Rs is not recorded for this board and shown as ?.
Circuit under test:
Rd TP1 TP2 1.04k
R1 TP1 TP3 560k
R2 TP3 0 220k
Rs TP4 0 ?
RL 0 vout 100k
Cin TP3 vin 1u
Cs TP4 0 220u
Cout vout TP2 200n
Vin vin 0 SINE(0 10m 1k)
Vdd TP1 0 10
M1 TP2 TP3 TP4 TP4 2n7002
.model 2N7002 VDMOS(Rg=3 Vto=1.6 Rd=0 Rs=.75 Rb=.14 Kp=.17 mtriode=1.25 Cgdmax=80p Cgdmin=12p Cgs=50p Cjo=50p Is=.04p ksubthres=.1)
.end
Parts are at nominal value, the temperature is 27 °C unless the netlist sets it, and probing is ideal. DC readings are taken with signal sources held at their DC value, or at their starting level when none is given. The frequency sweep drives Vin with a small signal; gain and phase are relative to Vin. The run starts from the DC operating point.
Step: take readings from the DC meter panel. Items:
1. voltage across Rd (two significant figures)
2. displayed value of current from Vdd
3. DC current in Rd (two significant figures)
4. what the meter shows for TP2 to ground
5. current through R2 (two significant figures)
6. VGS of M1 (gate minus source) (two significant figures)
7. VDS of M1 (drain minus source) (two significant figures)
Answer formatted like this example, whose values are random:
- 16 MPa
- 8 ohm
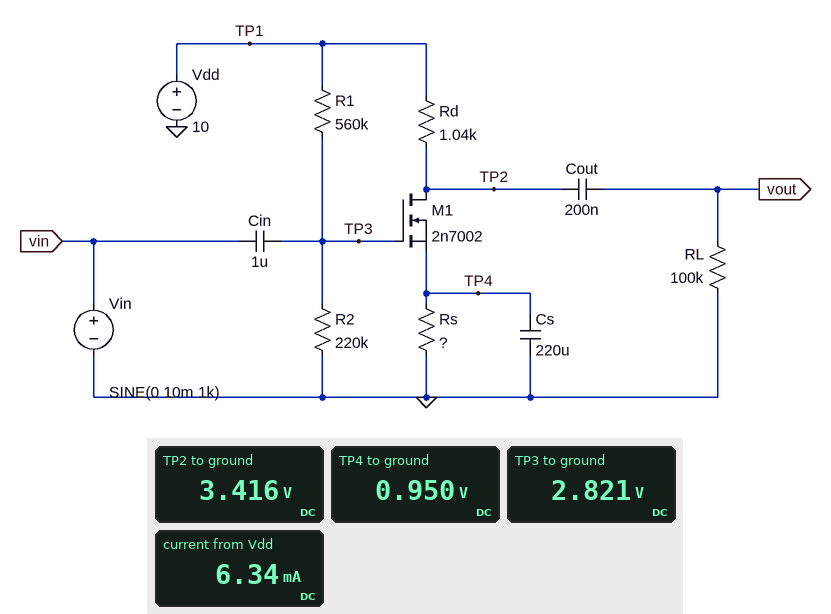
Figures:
- 6.6 V
- 6.34 mA
- 6.3 mA
- 3.416 V
- 13 µA
- 1.9 V
- 2.5 V
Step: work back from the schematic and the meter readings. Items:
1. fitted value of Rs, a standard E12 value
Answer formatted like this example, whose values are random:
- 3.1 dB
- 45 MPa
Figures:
- 150 Ω
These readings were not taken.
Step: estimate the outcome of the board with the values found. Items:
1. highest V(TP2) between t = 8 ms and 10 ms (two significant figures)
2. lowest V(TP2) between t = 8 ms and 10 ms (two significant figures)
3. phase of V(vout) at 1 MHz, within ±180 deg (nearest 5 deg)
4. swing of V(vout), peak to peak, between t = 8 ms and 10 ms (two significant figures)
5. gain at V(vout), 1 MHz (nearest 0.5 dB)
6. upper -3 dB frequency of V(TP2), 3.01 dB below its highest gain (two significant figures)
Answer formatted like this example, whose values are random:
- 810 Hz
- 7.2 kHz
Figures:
- 3.8 V
- 3.0 V
- 155 deg
- 860 mV
- 32.0 dB
- 2.2 MHz
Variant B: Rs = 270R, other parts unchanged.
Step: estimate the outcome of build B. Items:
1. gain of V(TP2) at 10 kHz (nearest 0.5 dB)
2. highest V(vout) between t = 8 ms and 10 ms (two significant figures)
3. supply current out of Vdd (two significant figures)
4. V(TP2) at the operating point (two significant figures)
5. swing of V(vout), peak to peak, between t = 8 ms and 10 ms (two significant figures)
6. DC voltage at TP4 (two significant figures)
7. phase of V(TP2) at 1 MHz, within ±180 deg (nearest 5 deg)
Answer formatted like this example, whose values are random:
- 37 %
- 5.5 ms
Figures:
- 30.0 dB
- 310 mV
- 3.8 mA
- 6.1 V
- 630 mV
- 1.0 V
- 165 deg
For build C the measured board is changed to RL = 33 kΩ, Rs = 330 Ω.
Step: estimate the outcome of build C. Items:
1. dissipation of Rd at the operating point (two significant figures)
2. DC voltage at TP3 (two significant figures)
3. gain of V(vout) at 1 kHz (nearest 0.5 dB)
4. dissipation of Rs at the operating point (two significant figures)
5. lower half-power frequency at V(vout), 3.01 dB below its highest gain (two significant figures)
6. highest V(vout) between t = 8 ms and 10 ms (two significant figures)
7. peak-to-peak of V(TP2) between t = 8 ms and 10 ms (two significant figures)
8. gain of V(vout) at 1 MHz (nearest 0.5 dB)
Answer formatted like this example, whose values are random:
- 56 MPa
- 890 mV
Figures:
- 10 mW
- 2.8 V
- 29.0 dB
- 3.3 mW
- 35 Hz
- 270 mV
- 550 mV
- 28.5 dB
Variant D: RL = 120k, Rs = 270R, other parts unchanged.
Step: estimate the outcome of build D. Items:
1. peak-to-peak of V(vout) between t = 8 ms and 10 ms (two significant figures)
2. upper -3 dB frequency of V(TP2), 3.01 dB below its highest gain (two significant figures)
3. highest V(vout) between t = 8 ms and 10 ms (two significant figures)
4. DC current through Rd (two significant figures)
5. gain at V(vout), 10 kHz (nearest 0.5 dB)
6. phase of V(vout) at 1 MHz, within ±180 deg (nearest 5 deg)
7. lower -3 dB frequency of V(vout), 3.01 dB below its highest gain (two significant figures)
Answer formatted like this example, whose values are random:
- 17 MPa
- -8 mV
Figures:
- 630 mV
- 3.8 MHz
- 310 mV
- 3.8 mA
- 30.0 dB
- 165 deg
- 26 Hz
